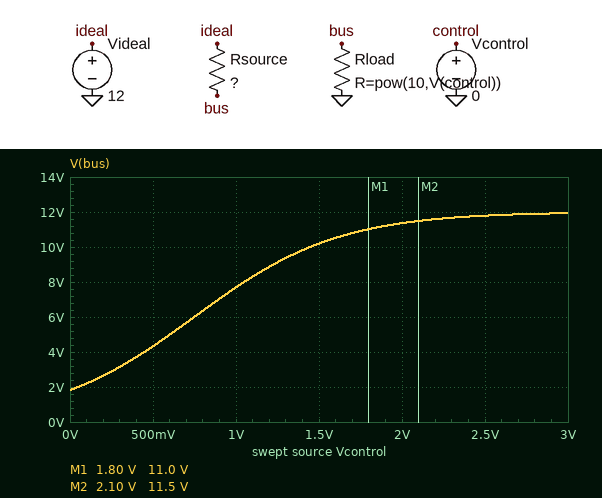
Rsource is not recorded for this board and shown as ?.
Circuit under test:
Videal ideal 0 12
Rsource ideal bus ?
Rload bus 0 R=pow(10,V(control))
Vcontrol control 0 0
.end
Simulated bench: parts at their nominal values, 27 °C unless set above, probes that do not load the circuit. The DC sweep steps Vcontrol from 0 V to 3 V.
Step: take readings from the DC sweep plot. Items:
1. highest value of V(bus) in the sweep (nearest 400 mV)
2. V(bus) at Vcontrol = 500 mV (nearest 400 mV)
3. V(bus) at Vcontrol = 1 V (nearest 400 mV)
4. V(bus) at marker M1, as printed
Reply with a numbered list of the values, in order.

1. 12.0 V
2. 4.4 V
3. 7.6 V
4. 11.0 V
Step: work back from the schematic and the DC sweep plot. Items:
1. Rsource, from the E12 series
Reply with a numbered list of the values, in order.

1. 5.6 Ω
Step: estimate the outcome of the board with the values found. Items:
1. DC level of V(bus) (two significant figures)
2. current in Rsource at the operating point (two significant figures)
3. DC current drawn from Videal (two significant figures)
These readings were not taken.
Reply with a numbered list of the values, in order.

1. 1.8 V
2. 1.8 A
3. 1.8 A
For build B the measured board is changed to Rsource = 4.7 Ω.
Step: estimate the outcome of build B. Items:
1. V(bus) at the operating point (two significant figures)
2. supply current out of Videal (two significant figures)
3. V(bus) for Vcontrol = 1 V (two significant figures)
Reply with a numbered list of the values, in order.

1. 2.1 V
2. 2.1 A
3. 8.2 V
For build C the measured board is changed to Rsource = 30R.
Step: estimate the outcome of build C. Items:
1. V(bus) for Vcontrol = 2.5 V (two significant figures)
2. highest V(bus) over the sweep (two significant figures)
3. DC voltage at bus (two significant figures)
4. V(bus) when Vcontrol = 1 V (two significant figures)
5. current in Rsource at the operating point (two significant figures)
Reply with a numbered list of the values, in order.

1. 11 V
2. 12 V
3. 390 mV
4. 3.0 V
5. 390 mA
